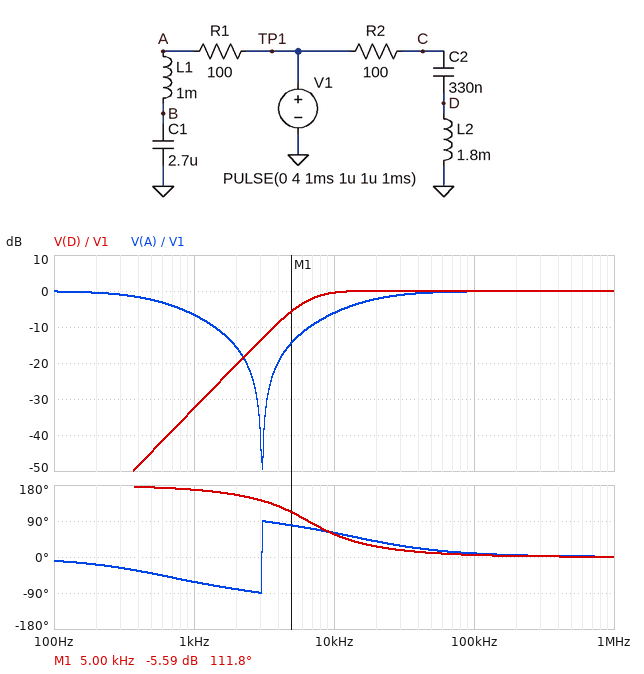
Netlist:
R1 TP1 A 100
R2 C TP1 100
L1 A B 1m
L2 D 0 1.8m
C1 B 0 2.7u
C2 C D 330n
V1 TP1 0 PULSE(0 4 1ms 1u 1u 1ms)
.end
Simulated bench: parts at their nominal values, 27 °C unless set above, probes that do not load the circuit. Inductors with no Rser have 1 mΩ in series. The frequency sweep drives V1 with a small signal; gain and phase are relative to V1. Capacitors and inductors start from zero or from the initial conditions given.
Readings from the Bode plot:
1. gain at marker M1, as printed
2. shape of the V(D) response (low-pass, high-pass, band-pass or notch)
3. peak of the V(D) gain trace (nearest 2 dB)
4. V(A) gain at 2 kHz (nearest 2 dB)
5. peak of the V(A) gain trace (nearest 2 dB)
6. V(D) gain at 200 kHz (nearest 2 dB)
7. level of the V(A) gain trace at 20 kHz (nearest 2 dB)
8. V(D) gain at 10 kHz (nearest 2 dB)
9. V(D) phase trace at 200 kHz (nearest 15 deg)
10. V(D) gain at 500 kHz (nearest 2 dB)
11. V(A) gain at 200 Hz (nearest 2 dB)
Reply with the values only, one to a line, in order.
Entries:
-5.59 dB
high-pass
0 dB
-16 dB
0 dB
0 dB
-2 dB
0 dB
0 deg
0 dB
0 dB
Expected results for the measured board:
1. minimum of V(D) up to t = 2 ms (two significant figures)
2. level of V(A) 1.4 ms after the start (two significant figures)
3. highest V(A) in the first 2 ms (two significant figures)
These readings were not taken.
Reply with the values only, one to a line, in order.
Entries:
-870 mV
3.1 V
3.9 V
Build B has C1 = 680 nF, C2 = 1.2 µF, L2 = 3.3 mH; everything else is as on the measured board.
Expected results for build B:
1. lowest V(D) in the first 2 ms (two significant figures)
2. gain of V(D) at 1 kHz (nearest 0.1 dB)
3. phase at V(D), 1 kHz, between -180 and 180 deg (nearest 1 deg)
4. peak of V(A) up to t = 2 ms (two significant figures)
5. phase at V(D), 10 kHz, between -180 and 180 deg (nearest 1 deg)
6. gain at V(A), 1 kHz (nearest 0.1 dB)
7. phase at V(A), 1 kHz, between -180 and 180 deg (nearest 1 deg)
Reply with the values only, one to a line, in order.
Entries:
-580 mV
-17.2 dB
138 deg
4.0 V
27 deg
-0.8 dB
-24 deg
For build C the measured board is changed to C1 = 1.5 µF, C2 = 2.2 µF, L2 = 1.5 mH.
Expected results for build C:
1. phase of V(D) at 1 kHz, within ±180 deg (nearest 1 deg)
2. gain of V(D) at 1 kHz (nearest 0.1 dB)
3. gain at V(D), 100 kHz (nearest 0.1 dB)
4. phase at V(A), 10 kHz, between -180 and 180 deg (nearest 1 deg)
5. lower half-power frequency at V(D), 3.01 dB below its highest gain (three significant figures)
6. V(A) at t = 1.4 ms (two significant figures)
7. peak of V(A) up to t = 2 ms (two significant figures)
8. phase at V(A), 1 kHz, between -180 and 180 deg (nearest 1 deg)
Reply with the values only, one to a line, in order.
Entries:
122 deg
-22.0 dB
0 dB
62 deg
9.89 kHz
3.7 V
4.0 V
-45 deg
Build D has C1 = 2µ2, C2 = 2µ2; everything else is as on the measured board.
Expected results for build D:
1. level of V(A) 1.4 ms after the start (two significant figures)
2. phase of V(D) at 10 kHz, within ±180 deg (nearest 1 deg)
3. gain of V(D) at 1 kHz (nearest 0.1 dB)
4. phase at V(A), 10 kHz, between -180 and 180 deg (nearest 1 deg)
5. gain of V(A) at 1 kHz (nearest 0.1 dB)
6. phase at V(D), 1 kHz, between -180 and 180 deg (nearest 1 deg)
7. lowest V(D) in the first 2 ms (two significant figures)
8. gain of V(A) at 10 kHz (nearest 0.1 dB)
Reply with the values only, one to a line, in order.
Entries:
3.3 V
43 deg
-20.3 dB
61 deg
-5.2 dB
121 deg
-240 mV
-6.3 dB
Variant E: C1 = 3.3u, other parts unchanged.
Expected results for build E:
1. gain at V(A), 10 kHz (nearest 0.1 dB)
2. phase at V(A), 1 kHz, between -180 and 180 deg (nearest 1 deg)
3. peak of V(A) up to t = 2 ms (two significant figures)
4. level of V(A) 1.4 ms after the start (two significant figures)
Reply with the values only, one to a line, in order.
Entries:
-6.0 dB
-67 deg
3.8 V
2.8 V
